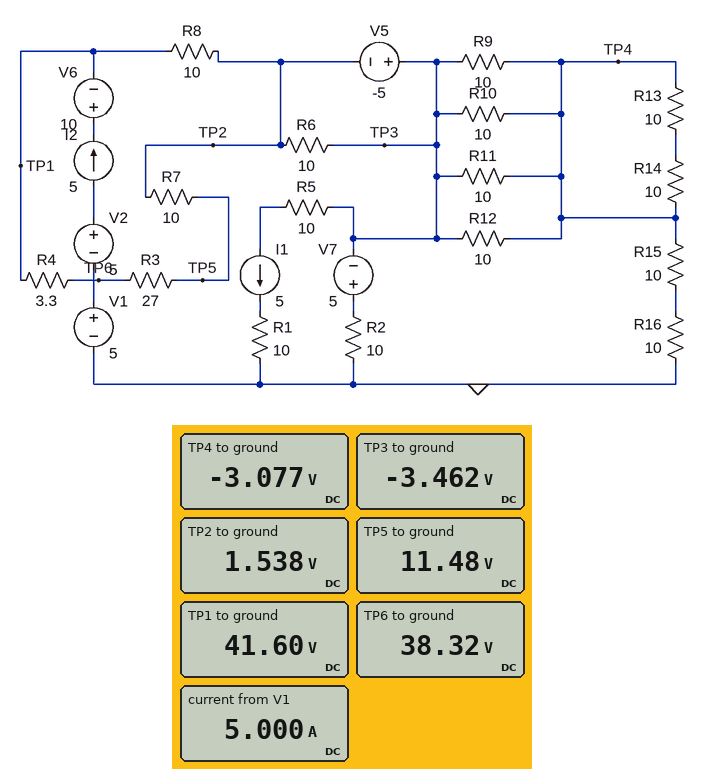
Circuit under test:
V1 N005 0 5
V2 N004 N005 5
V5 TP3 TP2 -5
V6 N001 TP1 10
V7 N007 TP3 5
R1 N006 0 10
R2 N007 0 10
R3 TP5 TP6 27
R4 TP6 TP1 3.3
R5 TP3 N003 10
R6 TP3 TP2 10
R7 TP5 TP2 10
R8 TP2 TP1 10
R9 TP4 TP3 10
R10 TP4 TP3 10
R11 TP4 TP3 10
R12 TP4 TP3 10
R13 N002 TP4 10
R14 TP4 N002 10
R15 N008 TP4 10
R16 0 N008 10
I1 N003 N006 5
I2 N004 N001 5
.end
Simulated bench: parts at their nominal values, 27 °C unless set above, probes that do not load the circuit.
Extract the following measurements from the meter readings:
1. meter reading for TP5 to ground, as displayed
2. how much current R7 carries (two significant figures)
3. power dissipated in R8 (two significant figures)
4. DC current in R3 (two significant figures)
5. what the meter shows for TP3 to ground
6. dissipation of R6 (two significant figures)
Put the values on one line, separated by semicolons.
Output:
11.48 V; 990 mA; 160 W; 990 mA; -3.462 V; 2.5 W
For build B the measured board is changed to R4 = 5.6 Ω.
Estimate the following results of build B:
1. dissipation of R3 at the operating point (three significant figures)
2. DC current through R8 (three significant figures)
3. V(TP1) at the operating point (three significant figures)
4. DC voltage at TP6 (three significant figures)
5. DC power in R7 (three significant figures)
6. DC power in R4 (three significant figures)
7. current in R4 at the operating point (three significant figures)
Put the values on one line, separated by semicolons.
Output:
24.4 W; 4.05 A; 42.0 V; 36.7 V; 9.04 W; 5.06 W; 951 mA
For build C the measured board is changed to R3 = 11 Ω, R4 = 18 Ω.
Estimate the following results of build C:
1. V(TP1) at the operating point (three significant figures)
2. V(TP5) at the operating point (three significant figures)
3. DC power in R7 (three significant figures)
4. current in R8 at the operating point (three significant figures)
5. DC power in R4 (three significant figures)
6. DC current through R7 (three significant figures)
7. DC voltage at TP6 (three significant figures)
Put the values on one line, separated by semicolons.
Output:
41.3 V; 11.7 V; 10.4 W; 3.98 A; 18.7 W; 1.02 A; 23.0 V
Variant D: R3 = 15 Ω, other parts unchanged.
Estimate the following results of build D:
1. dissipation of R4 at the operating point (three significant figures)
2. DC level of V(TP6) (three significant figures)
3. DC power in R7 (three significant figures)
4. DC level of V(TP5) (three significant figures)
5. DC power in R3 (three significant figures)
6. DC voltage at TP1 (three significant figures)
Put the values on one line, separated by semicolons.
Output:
5.62 W; 34.2 V; 17.0 W; 14.6 V; 25.6 W; 38.5 V
